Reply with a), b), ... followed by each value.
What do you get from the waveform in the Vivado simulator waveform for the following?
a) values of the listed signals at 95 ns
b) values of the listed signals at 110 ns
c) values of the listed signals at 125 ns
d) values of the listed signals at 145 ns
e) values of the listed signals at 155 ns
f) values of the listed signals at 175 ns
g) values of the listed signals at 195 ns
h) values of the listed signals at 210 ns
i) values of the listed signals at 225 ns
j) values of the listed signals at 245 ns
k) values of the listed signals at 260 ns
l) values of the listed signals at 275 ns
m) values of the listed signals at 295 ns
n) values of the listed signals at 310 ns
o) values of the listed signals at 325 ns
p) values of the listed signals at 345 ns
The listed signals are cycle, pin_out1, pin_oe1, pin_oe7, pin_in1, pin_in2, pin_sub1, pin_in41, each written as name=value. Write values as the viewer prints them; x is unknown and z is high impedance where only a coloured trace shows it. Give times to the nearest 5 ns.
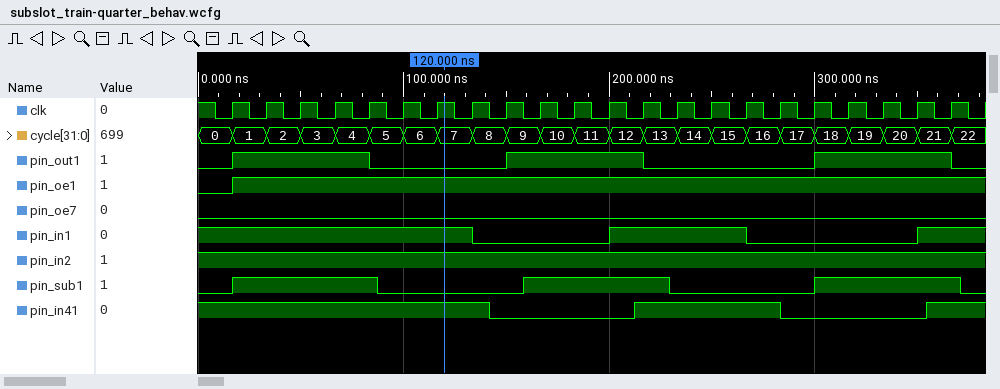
a) cycle=5, pin_out1=0, pin_oe1=1, pin_oe7=0, pin_in1=1, pin_in2=1, pin_sub1=0, pin_in41=1
b) cycle=6, pin_out1=0, pin_oe1=1, pin_oe7=0, pin_in1=1, pin_in2=1, pin_sub1=0, pin_in41=1
c) cycle=7, pin_out1=0, pin_oe1=1, pin_oe7=0, pin_in1=1, pin_in2=1, pin_sub1=0, pin_in41=1
d) cycle=8, pin_out1=0, pin_oe1=1, pin_oe7=0, pin_in1=0, pin_in2=1, pin_sub1=0, pin_in41=0
e) cycle=9, pin_out1=1, pin_oe1=1, pin_oe7=0, pin_in1=0, pin_in2=1, pin_sub1=0, pin_in41=0
f) cycle=10, pin_out1=1, pin_oe1=1, pin_oe7=0, pin_in1=0, pin_in2=1, pin_sub1=1, pin_in41=0
g) cycle=11, pin_out1=1, pin_oe1=1, pin_oe7=0, pin_in1=0, pin_in2=1, pin_sub1=1, pin_in41=0
h) cycle=12, pin_out1=1, pin_oe1=1, pin_oe7=0, pin_in1=1, pin_in2=1, pin_sub1=1, pin_in41=0
i) cycle=13, pin_out1=0, pin_oe1=1, pin_oe7=0, pin_in1=1, pin_in2=1, pin_sub1=1, pin_in41=1
j) cycle=14, pin_out1=0, pin_oe1=1, pin_oe7=0, pin_in1=1, pin_in2=1, pin_sub1=0, pin_in41=1
k) cycle=15, pin_out1=0, pin_oe1=1, pin_oe7=0, pin_in1=1, pin_in2=1, pin_sub1=0, pin_in41=1
l) cycle=16, pin_out1=0, pin_oe1=1, pin_oe7=0, pin_in1=0, pin_in2=1, pin_sub1=0, pin_in41=1
m) cycle=17, pin_out1=0, pin_oe1=1, pin_oe7=0, pin_in1=0, pin_in2=1, pin_sub1=0, pin_in41=0
n) cycle=18, pin_out1=1, pin_oe1=1, pin_oe7=0, pin_in1=0, pin_in2=1, pin_sub1=1, pin_in41=0
o) cycle=19, pin_out1=1, pin_oe1=1, pin_oe7=0, pin_in1=0, pin_in2=1, pin_sub1=1, pin_in41=0
p) cycle=20, pin_out1=1, pin_oe1=1, pin_oe7=0, pin_in1=0, pin_in2=1, pin_sub1=1, pin_in41=0
